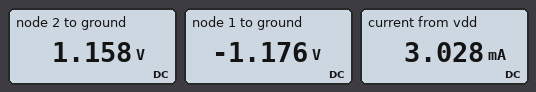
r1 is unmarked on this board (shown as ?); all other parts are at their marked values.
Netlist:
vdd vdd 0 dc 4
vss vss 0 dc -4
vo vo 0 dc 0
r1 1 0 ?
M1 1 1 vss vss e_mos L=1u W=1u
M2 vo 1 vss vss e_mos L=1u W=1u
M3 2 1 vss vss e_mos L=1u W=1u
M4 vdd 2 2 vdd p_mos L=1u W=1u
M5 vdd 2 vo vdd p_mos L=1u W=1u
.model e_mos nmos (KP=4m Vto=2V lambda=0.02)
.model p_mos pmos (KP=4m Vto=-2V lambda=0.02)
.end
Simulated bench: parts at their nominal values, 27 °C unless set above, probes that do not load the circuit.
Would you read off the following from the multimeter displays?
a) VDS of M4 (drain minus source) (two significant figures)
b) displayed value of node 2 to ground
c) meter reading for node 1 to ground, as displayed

2.8 V
1.158 V
-1.176 V
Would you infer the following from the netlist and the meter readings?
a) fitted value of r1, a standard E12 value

820 Ω
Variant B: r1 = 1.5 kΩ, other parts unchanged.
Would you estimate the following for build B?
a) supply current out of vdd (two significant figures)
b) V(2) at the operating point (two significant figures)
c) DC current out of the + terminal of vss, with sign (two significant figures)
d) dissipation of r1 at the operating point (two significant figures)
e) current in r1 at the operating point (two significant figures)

1.9 mA
1.3 V
-2.8 mA
1.2 mW
900 µA
